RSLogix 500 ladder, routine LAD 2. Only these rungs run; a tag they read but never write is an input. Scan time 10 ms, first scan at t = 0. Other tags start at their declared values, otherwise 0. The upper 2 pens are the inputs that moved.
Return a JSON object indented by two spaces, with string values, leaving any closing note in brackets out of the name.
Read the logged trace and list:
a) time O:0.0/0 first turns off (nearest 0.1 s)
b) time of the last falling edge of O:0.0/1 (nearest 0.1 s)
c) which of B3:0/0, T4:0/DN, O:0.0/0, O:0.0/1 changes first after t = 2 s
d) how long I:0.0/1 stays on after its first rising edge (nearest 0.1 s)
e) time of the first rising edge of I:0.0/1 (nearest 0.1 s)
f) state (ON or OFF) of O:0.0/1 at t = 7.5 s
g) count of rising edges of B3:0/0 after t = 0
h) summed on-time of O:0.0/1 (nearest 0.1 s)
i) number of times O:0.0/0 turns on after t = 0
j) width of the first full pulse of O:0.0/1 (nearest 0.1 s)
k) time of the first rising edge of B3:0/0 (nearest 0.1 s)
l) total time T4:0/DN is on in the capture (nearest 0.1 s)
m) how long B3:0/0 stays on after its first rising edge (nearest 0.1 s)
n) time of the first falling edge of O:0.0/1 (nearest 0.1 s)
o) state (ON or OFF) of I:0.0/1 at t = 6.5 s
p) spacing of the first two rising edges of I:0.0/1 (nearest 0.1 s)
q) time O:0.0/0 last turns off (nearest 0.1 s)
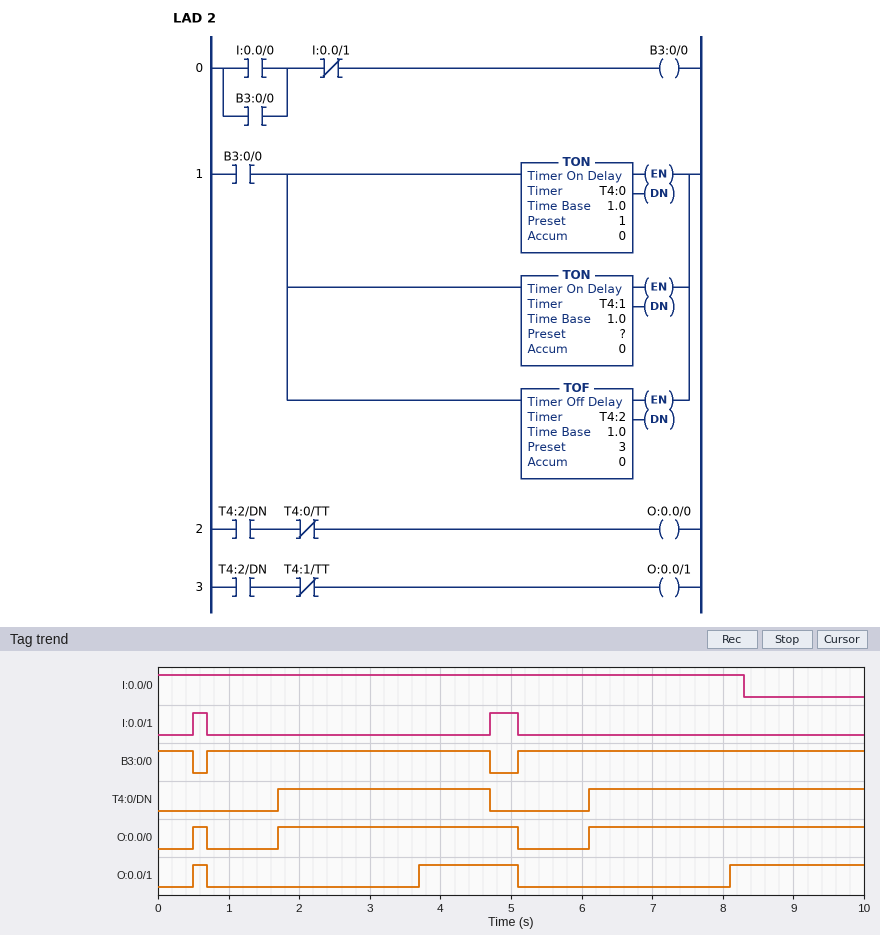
{
  "time O:0.0/0 first turns off": "0.7 s",
  "time of the last falling edge of O:0.0/1": "5.1 s",
  "which of B3:0/0, T4:0/DN, O:0.0/0, O:0.0/1 changes first after t = 2 s": "O:0.0/1",
  "how long I:0.0/1 stays on after its first rising edge": "0.2 s",
  "time of the first rising edge of I:0.0/1": "0.5 s",
  "state (ON or OFF) of O:0.0/1 at t = 7.5 s": "OFF",
  "count of rising edges of B3:0/0 after t = 0": "2",
  "summed on-time of O:0.0/1": "3.5 s",
  "number of times O:0.0/0 turns on after t = 0": "3",
  "width of the first full pulse of O:0.0/1": "0.2 s",
  "time of the first rising edge of B3:0/0": "0.7 s",
  "total time T4:0/DN is on in the capture": "6.9 s",
  "how long B3:0/0 stays on after its first rising edge": "4.0 s",
  "time of the first falling edge of O:0.0/1": "0.7 s",
  "state (ON or OFF) of I:0.0/1 at t = 6.5 s": "OFF",
  "spacing of the first two rising edges of I:0.0/1": "4.2 s",
  "time O:0.0/0 last turns off": "5.1 s"
}
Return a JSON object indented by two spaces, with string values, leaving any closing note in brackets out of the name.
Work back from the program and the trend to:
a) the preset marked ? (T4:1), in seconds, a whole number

{
  "the preset marked ? (T4:1), in seconds, a whole number": "3 s"
}
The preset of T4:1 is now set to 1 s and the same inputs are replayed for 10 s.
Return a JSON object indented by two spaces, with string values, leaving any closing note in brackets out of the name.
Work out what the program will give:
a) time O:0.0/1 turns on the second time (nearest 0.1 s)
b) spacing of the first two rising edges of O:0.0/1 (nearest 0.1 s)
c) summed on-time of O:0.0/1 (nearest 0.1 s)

{
  "time O:0.0/1 turns on the second time": "1.7 s",
  "spacing of the first two rising edges of O:0.0/1": "1.2 s",
  "summed on-time of O:0.0/1": "7.5 s"
}
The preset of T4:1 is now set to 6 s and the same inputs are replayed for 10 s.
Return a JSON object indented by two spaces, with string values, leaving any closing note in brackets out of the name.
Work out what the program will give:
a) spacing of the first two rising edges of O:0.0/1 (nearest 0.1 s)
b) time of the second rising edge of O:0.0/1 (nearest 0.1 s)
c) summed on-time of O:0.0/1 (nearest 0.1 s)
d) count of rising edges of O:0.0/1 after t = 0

{
  "spacing of the first two rising edges of O:0.0/1": "4.2 s",
  "time of the second rising edge of O:0.0/1": "4.7 s",
  "summed on-time of O:0.0/1": "0.6 s",
  "count of rising edges of O:0.0/1 after t = 0": "2"
}
